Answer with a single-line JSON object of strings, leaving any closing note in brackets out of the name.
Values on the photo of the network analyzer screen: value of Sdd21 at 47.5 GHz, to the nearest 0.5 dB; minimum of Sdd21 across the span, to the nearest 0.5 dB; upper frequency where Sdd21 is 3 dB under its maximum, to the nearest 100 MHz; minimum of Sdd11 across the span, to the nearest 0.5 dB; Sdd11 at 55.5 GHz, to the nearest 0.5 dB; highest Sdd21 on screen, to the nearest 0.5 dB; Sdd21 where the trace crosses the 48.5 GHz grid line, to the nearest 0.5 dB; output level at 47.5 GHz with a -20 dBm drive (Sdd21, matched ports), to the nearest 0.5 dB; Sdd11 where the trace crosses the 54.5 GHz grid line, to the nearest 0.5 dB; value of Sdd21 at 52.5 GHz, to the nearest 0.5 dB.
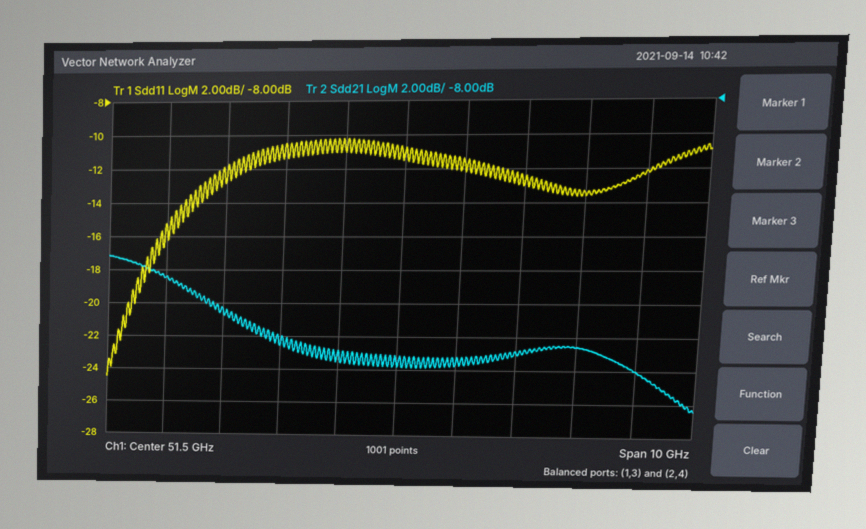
{"value of Sdd21 at 47.5 GHz, to the nearest 0.5 dB": "-18.5 dB", "minimum of Sdd21 across the span, to the nearest 0.5 dB": "-26.5 dB", "upper frequency where Sdd21 is 3 dB under its maximum, to the nearest 100 MHz": "48.3 GHz", "minimum of Sdd11 across the span, to the nearest 0.5 dB": "-24.5 dB", "Sdd11 at 55.5 GHz, to the nearest 0.5 dB": "-12.0 dB", "highest Sdd21 on screen, to the nearest 0.5 dB": "-17.0 dB", "Sdd21 where the trace crosses the 48.5 GHz grid line, to the nearest 0.5 dB": "-20.5 dB", "output level at 47.5 GHz with a -20 dBm drive (Sdd21, matched ports), to the nearest 0.5 dB": "-38.5 dBm", "Sdd11 where the trace crosses the 54.5 GHz grid line, to the nearest 0.5 dB": "-13.5 dB", "value of Sdd21 at 52.5 GHz, to the nearest 0.5 dB": "-23.5 dB"}
